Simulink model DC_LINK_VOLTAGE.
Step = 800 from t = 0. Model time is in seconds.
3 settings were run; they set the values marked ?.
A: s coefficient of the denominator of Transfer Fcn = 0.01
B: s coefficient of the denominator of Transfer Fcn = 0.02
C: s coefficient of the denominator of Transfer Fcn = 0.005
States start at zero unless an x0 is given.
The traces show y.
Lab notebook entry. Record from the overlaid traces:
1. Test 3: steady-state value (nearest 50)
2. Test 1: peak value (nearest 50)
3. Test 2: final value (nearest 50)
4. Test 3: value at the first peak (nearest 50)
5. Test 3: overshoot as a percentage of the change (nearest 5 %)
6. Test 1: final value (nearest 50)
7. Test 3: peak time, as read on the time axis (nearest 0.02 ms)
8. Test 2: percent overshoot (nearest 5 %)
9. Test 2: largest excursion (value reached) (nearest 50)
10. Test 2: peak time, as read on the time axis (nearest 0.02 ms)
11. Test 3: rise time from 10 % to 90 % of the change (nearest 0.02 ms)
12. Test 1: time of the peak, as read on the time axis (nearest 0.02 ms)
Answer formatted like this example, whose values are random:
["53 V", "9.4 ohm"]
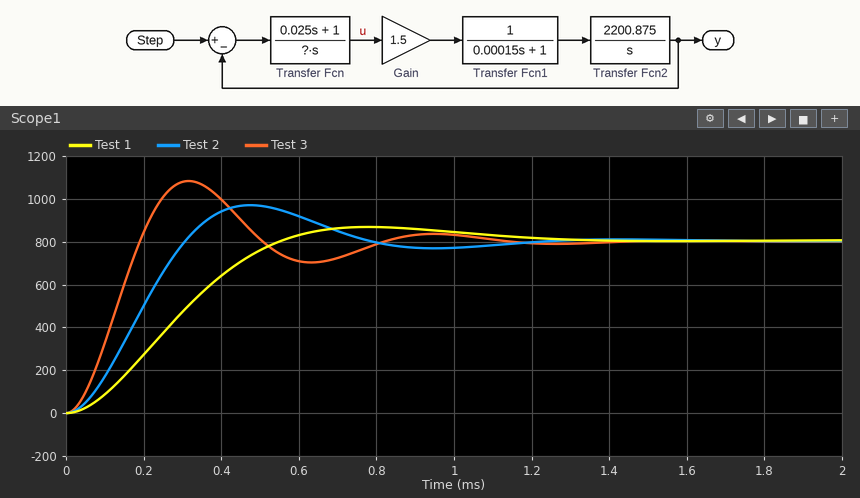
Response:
["800", "850", "800", "1100", "35 %", "800", "0.32 ms", "20 %", "950", "0.48 ms", "0.12 ms", "0.78 ms"]
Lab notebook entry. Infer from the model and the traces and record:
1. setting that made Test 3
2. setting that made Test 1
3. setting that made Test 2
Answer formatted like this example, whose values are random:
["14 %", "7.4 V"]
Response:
["C", "B", "A"]
